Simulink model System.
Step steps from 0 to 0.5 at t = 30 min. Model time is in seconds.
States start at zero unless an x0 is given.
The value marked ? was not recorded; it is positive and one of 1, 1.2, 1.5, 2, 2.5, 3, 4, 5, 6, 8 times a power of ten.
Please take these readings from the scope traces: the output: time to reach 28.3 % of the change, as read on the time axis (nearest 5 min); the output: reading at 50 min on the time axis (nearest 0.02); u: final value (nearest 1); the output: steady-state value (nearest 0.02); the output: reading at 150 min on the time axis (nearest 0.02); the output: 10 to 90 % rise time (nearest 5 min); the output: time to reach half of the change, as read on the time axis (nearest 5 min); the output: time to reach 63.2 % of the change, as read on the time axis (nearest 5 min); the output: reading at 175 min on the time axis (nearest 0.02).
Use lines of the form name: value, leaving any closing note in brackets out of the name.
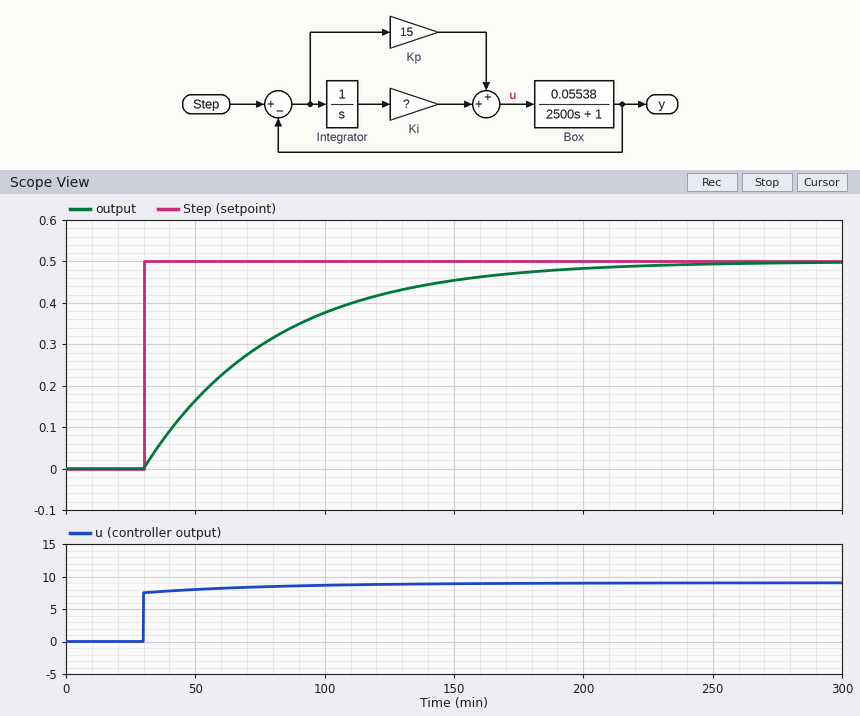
the output: time to reach 28.3 % of the change, as read on the time axis: 45 min
the output: reading at 50 min on the time axis: 0.16
u: final value: 9
the output: steady-state value: 0.50
the output: reading at 150 min on the time axis: 0.46
the output: 10 to 90 % rise time: 110 min
the output: time to reach half of the change, as read on the time axis: 65 min
the output: time to reach 63.2 % of the change, as read on the time axis: 80 min
the output: reading at 175 min on the time axis: 0.48
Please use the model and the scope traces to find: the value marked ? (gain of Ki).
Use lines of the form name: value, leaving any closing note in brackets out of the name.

the value marked ?: 0.006
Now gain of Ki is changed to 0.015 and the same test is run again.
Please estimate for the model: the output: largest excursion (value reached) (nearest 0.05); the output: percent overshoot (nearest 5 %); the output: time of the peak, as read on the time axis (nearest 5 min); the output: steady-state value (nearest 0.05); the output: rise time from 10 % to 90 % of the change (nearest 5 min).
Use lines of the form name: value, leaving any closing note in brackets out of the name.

the output: largest excursion (value reached): 0.55
the output: percent overshoot: 10 %
the output: time of the peak, as read on the time axis: 125 min
the output: steady-state value: 0.50
the output: rise time from 10 % to 90 % of the change: 45 min
